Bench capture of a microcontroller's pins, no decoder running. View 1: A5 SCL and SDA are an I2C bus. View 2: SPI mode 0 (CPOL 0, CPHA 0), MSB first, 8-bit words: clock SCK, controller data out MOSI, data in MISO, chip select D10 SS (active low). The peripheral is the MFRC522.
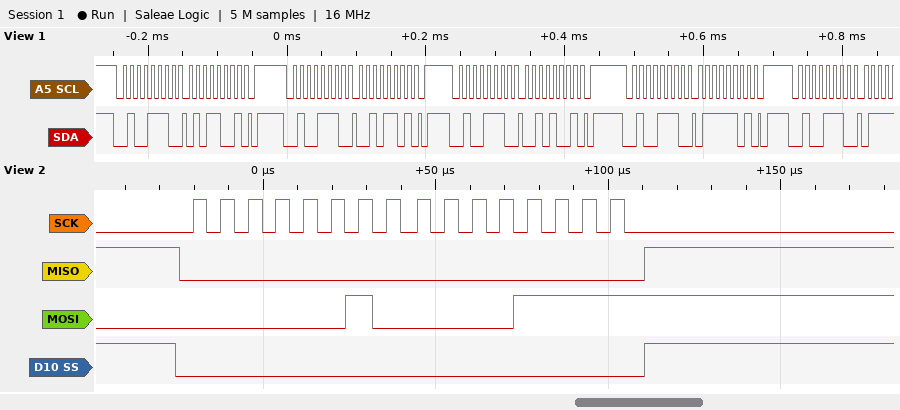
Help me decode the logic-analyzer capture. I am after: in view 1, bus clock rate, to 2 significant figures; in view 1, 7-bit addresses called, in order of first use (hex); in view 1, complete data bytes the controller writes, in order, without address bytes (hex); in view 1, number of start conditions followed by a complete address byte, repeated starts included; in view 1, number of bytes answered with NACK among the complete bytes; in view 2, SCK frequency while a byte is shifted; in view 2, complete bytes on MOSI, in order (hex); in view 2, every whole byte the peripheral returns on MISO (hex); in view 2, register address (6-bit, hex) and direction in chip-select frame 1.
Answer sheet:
100 kHz
0x27
59 2D 29 7D
5
0
125 kHz
0x02 0x0F
0x00 0x00
0x01 write
